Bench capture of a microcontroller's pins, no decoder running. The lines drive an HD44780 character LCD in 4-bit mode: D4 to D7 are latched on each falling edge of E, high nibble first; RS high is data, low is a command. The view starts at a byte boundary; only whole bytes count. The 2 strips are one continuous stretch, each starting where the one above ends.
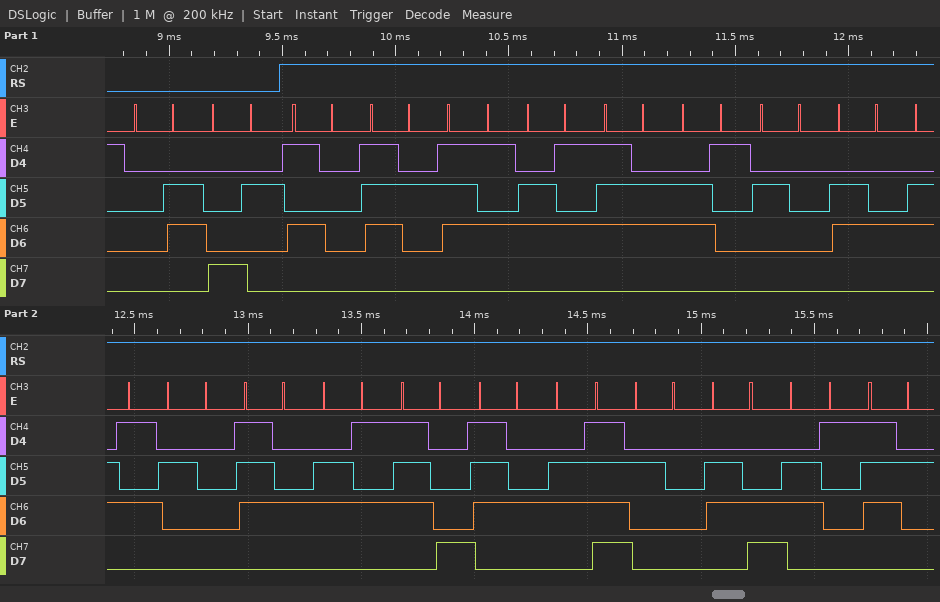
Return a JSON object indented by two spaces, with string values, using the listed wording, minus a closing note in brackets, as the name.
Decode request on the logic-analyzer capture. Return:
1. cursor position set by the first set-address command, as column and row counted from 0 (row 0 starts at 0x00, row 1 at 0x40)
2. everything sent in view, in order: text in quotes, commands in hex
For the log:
{
  "cursor position set by the first set-address command, as column and row counted from 0": "column 2, row 0",
  "everything sent in view, in order: text in quotes, commands in hex": "0x06 0x82 \"Prueva de texto lar\""
}
